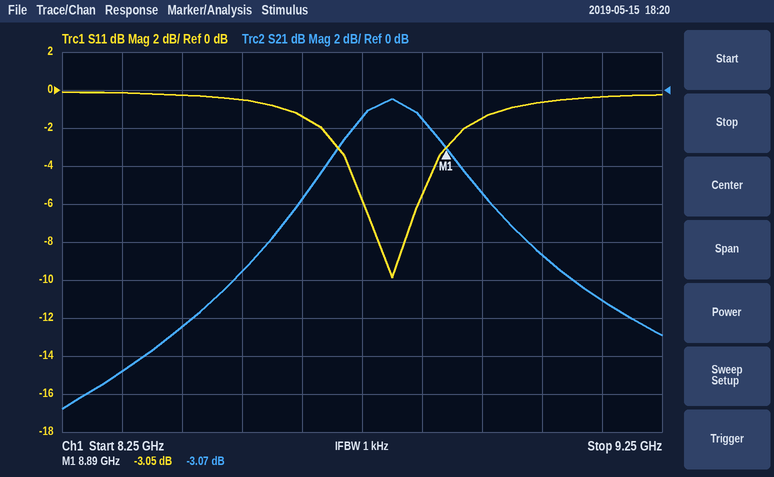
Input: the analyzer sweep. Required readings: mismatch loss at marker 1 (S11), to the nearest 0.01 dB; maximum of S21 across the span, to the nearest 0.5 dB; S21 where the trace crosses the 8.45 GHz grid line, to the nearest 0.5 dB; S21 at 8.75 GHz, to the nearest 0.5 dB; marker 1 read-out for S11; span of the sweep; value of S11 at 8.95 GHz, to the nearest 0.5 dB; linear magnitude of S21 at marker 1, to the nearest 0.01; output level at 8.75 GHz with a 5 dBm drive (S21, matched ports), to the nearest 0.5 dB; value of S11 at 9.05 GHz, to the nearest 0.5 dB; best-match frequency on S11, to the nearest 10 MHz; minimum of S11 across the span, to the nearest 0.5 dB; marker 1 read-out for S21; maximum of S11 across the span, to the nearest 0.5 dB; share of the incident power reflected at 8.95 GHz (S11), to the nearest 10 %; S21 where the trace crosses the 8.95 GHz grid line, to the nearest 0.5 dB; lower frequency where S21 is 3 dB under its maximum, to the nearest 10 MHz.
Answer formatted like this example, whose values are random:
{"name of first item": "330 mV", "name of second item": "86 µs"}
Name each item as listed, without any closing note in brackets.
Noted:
{"mismatch loss at marker 1 (S11), to the nearest 0.01 dB": "2.97 dB", "maximum of S21 across the span, to the nearest 0.5 dB": "-0.5 dB", "S21 where the trace crosses the 8.45 GHz grid line, to the nearest 0.5 dB": "-12.5 dB", "S21 at 8.75 GHz, to the nearest 0.5 dB": "-1.5 dB", "marker 1 read-out for S11": "-3.05 dB", "span of the sweep": "1 GHz", "value of S11 at 8.95 GHz, to the nearest 0.5 dB": "-1.5 dB", "linear magnitude of S21 at marker 1, to the nearest 0.01": "0.70", "output level at 8.75 GHz with a 5 dBm drive (S21, matched ports), to the nearest 0.5 dB": "3.5 dBm", "value of S11 at 9.05 GHz, to the nearest 0.5 dB": "-0.5 dB", "best-match frequency on S11, to the nearest 10 MHz": "8.80 GHz", "minimum of S11 across the span, to the nearest 0.5 dB": "-10.0 dB", "marker 1 read-out for S21": "-3.07 dB", "maximum of S11 across the span, to the nearest 0.5 dB": "0.0 dB", "share of the incident power reflected at 8.95 GHz (S11), to the nearest 10 %": "70 %", "S21 where the trace crosses the 8.95 GHz grid line, to the nearest 0.5 dB": "-5.5 dB", "lower frequency where S21 is 3 dB under its maximum, to the nearest 10 MHz": "8.70 GHz"}
